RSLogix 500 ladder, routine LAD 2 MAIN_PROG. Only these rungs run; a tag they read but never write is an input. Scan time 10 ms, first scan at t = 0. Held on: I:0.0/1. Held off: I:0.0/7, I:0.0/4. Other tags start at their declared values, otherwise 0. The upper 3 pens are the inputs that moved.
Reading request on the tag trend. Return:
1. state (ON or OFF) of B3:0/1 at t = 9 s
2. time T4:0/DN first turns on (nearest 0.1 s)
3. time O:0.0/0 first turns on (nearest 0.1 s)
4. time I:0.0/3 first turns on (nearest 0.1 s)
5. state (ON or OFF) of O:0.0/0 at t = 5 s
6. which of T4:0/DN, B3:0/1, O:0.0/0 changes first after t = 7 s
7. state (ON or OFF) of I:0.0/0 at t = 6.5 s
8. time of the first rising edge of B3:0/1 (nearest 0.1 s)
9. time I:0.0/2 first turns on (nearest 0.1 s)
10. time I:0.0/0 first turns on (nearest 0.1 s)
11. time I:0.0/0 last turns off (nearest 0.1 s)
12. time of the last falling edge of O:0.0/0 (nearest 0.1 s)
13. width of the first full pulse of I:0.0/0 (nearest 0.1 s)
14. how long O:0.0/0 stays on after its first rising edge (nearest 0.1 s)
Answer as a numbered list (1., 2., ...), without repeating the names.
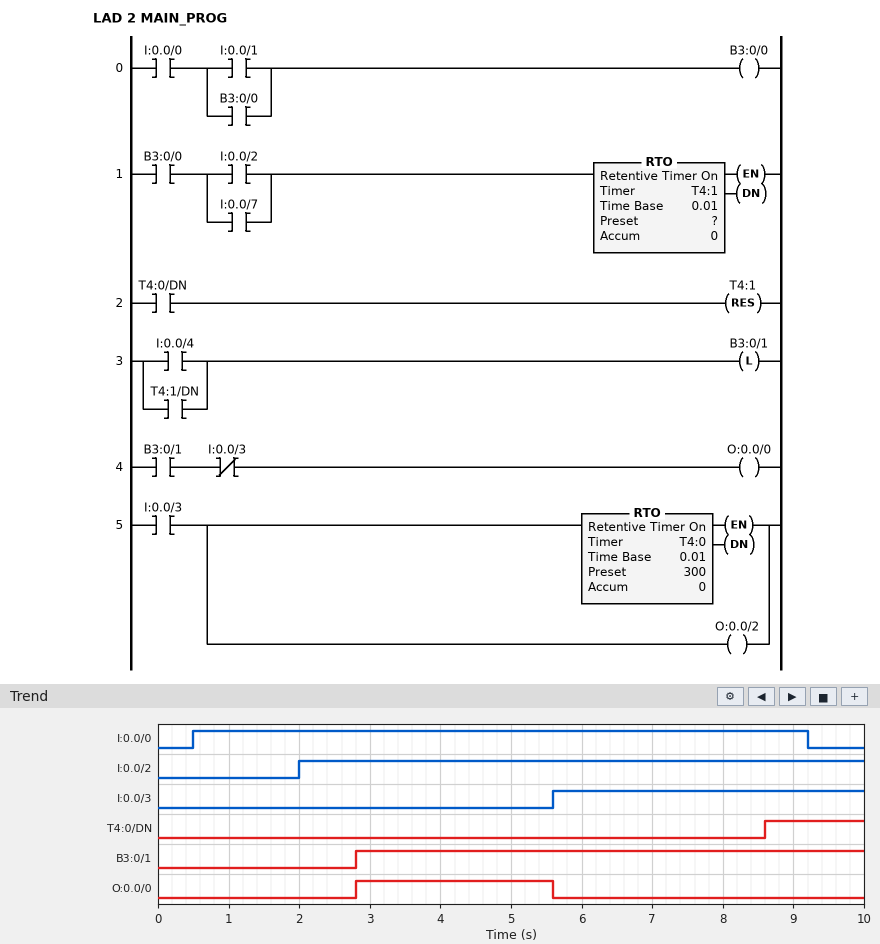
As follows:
1. ON
2. 8.6 s
3. 2.8 s
4. 5.6 s
5. ON
6. T4:0/DN
7. ON
8. 2.8 s
9. 2.0 s
10. 0.5 s
11. 9.2 s
12. 5.6 s
13. 8.7 s
14. 2.8 s
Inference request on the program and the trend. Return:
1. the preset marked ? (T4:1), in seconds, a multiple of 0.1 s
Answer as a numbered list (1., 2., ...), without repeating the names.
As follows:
1. 0.8 s
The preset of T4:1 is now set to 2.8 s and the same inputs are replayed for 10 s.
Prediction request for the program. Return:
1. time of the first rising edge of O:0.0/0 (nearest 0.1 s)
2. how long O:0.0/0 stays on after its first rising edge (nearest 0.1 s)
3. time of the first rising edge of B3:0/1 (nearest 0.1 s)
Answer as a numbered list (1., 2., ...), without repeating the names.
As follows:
1. 4.8 s
2. 0.8 s
3. 4.8 s
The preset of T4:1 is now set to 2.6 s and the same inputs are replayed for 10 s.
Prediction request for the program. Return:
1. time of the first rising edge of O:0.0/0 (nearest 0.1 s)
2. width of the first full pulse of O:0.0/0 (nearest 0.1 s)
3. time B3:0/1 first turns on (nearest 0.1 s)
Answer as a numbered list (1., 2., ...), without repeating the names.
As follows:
1. 4.6 s
2. 1.0 s
3. 4.6 s
